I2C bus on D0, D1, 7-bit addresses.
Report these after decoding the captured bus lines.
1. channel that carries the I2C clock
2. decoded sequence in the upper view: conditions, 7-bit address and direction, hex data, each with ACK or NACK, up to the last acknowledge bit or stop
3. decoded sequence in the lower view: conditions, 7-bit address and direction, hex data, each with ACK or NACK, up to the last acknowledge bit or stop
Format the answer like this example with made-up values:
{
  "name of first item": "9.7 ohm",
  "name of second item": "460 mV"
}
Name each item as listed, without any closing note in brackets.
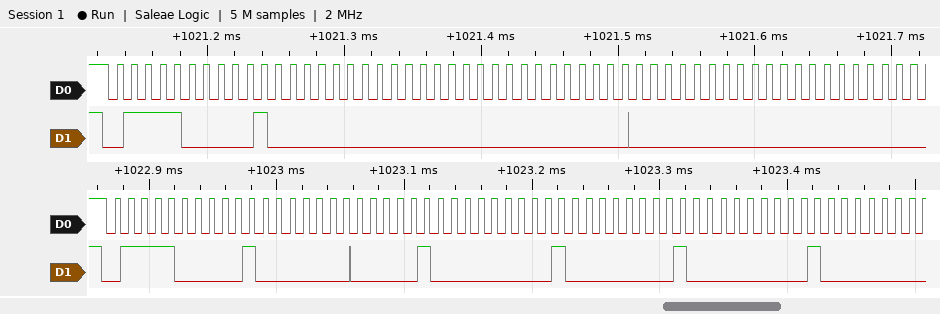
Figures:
{
  "channel that carries the I2C clock": "D0",
  "decoded sequence in the upper view: conditions, 7-bit address and direction, hex data, each with ACK or NACK, up to the last acknowledge bit or stop": "start, address 3C write ACK, 40 ACK, 00 ACK, 00 ACK, 00 ACK, 00 ACK",
  "decoded sequence in the lower view: conditions, 7-bit address and direction, hex data, each with ACK or NACK, up to the last acknowledge bit or stop": "start, address 3C write ACK, 40 ACK, 04 ACK, 02 ACK, 02 ACK, 01 ACK"
}
